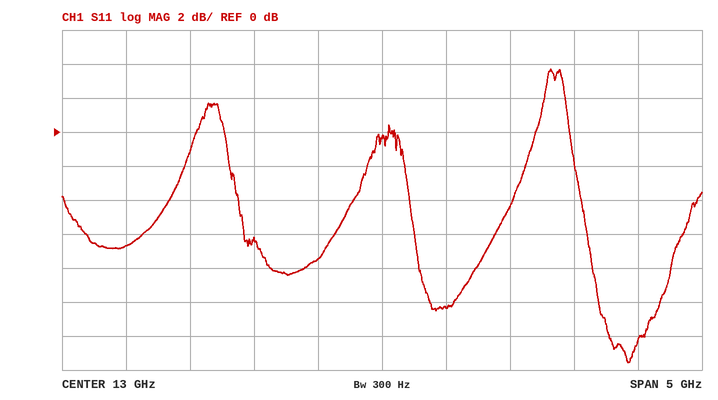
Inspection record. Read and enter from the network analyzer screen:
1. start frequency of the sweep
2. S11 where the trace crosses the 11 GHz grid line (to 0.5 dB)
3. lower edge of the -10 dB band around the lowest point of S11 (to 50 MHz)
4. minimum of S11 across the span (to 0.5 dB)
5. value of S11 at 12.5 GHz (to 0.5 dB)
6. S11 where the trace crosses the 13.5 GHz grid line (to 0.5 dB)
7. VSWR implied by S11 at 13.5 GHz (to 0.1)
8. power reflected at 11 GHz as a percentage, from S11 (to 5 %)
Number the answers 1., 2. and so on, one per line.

1. 10.5 GHz
2. -6.5 dB
3. 14.70 GHz
4. -13.5 dB
5. -7.5 dB
6. -10.5 dB
7. 1.9
8. 20 %
